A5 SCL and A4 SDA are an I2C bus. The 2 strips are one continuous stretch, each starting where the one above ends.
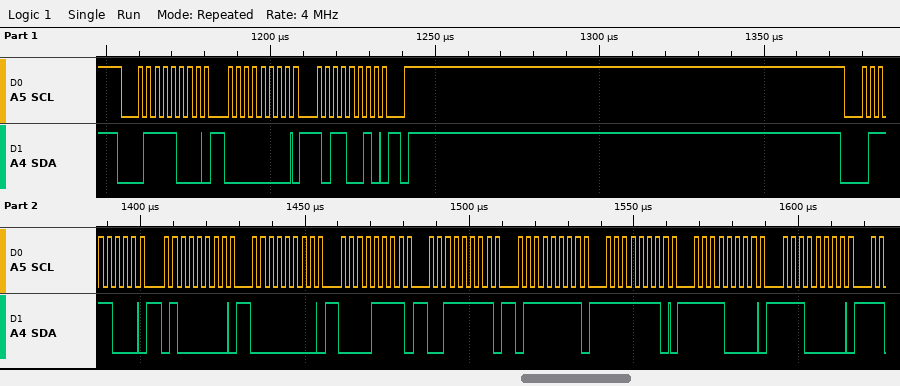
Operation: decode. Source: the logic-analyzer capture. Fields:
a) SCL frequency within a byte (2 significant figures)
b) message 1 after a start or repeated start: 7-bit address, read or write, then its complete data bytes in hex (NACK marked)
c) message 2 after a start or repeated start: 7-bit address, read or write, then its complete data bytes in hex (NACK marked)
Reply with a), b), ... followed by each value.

a) 400 kHz
b) 0x3C write: 00 B2
c) 0x3C write: 40 00 0F 3F 7F FE F0 E0
